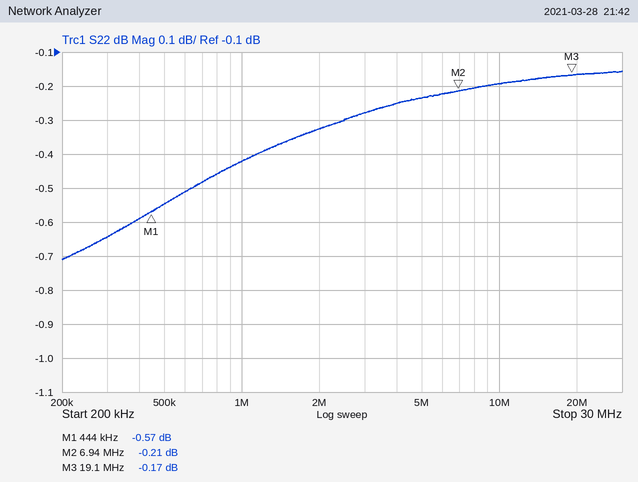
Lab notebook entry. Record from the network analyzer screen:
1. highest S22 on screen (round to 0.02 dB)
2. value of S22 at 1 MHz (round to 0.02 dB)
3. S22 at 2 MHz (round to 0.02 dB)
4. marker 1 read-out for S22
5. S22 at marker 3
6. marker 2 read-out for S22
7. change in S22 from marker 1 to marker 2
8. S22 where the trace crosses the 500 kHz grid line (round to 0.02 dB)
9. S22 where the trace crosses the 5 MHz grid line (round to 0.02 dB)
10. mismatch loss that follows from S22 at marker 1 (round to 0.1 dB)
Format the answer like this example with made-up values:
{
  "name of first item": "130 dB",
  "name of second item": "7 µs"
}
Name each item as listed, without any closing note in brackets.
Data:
{
  "highest S22 on screen": "-0.16 dB",
  "value of S22 at 1 MHz": "-0.42 dB",
  "S22 at 2 MHz": "-0.32 dB",
  "marker 1 read-out for S22": "-0.57 dB",
  "S22 at marker 3": "-0.17 dB",
  "marker 2 read-out for S22": "-0.21 dB",
  "change in S22 from marker 1 to marker 2": "0.36 dB",
  "S22 where the trace crosses the 500 kHz grid line": "-0.54 dB",
  "S22 where the trace crosses the 5 MHz grid line": "-0.24 dB",
  "mismatch loss that follows from S22 at marker 1": "9.1 dB"
}
